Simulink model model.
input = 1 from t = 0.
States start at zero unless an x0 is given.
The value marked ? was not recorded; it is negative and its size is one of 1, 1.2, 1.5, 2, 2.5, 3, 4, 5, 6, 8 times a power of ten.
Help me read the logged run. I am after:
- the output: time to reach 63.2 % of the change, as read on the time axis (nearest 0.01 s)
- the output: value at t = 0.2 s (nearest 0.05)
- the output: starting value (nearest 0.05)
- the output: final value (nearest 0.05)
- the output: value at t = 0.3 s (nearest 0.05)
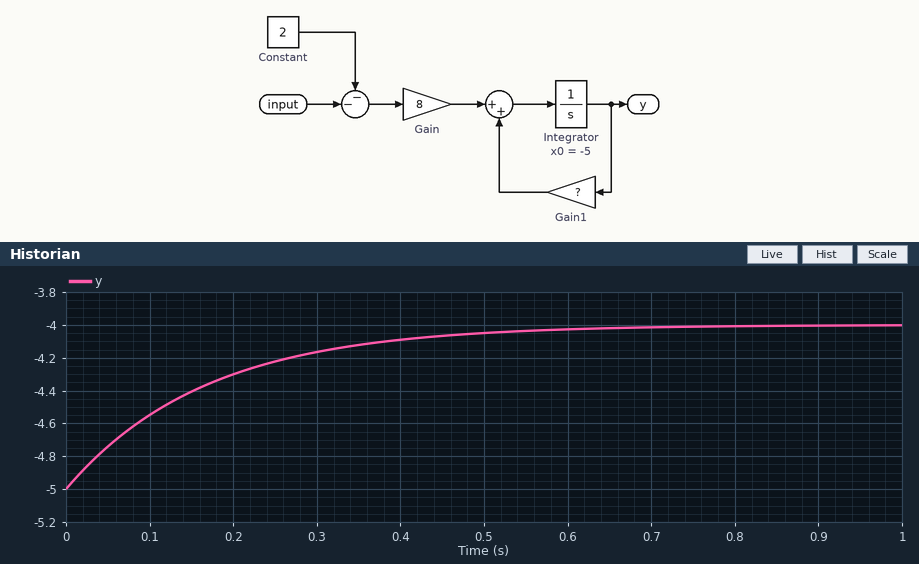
0.17 s
-4.30
-5.00
-4.00
-4.15
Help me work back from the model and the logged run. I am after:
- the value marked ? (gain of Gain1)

-6
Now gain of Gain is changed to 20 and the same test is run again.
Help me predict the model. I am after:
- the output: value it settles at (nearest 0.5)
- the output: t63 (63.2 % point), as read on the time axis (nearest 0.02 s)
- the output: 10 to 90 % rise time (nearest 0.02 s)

-10.0
0.16 s
0.36 s
